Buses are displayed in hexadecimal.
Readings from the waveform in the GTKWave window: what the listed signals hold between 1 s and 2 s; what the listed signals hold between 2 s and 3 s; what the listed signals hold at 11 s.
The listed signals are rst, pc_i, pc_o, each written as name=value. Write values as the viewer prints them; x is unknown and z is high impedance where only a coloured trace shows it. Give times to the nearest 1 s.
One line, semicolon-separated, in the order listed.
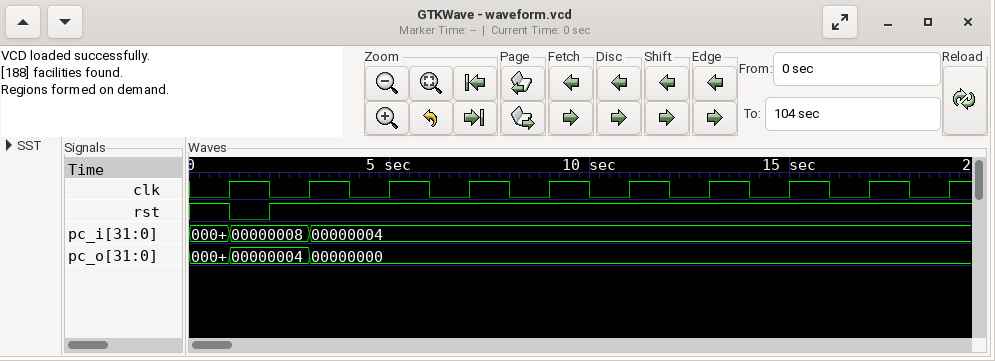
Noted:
rst=0, pc_i=00000008, pc_o=00000004; rst=1, pc_i=00000008, pc_o=00000004; rst=1, pc_i=00000004, pc_o=00000000
